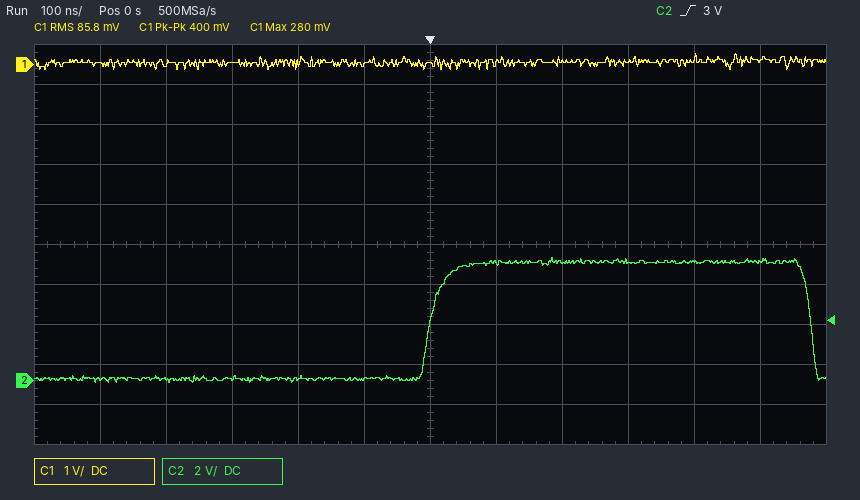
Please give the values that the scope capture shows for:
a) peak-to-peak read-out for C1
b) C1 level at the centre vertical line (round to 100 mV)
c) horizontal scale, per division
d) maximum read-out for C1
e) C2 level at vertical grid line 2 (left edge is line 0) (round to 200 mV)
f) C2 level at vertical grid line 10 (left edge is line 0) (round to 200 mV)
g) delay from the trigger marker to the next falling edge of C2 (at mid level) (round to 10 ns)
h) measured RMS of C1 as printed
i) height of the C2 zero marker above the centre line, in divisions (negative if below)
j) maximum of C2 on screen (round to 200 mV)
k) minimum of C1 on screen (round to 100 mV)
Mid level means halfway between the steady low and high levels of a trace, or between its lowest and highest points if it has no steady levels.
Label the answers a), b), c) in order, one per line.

a) 400 mV
b) 0.0 V
c) 100 ns
d) 280 mV
e) 0.0 V
f) 6.0 V
g) 580 ns
h) 85.8 mV
i) -3.4 div
j) 6.2 V
k) -100 mV
